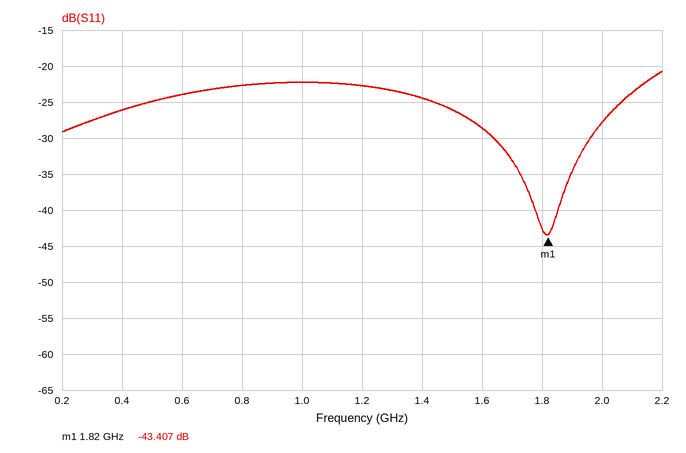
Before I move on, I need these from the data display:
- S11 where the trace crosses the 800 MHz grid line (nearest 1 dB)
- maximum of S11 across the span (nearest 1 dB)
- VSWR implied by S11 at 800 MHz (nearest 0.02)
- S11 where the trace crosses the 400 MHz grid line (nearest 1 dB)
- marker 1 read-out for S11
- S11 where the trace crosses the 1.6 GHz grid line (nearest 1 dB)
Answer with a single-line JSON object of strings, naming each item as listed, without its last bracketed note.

{"S11 where the trace crosses the 800 MHz grid line": "-23 dB", "maximum of S11 across the span": "-21 dB", "VSWR implied by S11 at 800 MHz": "1.16", "S11 where the trace crosses the 400 MHz grid line": "-26 dB", "marker 1 read-out for S11": "-43.407 dB", "S11 where the trace crosses the 1.6 GHz grid line": "-29 dB"}
